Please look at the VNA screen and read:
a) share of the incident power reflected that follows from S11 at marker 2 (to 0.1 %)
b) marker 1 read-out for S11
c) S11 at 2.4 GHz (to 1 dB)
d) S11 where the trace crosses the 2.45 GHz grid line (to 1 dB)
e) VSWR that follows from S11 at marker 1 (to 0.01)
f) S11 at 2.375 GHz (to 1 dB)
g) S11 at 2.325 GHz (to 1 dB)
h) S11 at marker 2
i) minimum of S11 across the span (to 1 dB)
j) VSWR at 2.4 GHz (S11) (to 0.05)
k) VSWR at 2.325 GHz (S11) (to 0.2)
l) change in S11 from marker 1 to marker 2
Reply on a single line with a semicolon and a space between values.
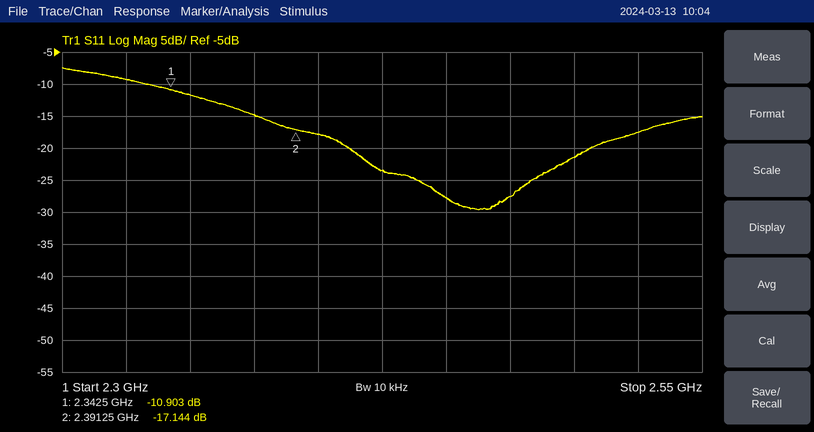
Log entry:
1.9 %; -10.903 dB; -18 dB; -28 dB; 1.80; -15 dB; -9 dB; -17.144 dB; -30 dB; 1.30; 2.0; -6.241 dB
